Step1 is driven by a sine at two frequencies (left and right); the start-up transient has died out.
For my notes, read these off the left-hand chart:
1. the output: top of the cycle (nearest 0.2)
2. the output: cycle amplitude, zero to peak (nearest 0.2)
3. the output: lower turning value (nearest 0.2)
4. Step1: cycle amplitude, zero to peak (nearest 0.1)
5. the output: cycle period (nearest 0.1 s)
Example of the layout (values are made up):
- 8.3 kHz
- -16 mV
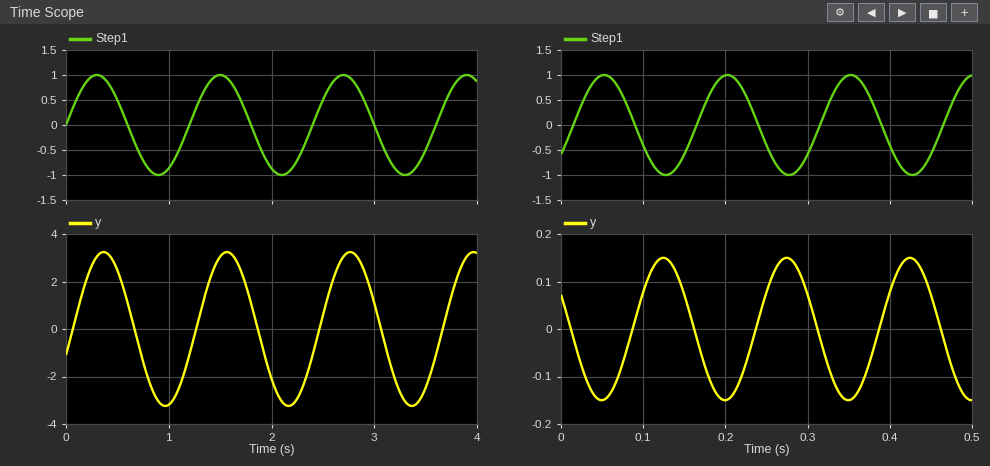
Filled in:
- 3.2
- 3.2
- -3.2
- 1.0
- 1.2 s
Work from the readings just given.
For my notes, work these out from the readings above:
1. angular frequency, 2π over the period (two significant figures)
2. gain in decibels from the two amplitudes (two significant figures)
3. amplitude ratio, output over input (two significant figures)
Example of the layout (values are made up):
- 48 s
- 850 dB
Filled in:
- 5.2 rad/s
- 10 dB
- 3.2
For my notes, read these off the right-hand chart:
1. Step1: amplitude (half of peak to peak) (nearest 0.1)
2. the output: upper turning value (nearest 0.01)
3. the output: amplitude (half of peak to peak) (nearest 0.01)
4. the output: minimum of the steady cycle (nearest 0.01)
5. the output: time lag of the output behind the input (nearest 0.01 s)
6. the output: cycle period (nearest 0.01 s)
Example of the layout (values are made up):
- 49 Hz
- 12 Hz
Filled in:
- 1.0
- 0.15
- 0.15
- -0.15
- 0.07 s
- 0.15 s
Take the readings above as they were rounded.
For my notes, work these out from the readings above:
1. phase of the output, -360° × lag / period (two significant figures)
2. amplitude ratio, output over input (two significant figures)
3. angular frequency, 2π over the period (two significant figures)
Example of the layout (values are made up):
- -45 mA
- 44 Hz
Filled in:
- -170°
- 0.15
- 42 rad/s
